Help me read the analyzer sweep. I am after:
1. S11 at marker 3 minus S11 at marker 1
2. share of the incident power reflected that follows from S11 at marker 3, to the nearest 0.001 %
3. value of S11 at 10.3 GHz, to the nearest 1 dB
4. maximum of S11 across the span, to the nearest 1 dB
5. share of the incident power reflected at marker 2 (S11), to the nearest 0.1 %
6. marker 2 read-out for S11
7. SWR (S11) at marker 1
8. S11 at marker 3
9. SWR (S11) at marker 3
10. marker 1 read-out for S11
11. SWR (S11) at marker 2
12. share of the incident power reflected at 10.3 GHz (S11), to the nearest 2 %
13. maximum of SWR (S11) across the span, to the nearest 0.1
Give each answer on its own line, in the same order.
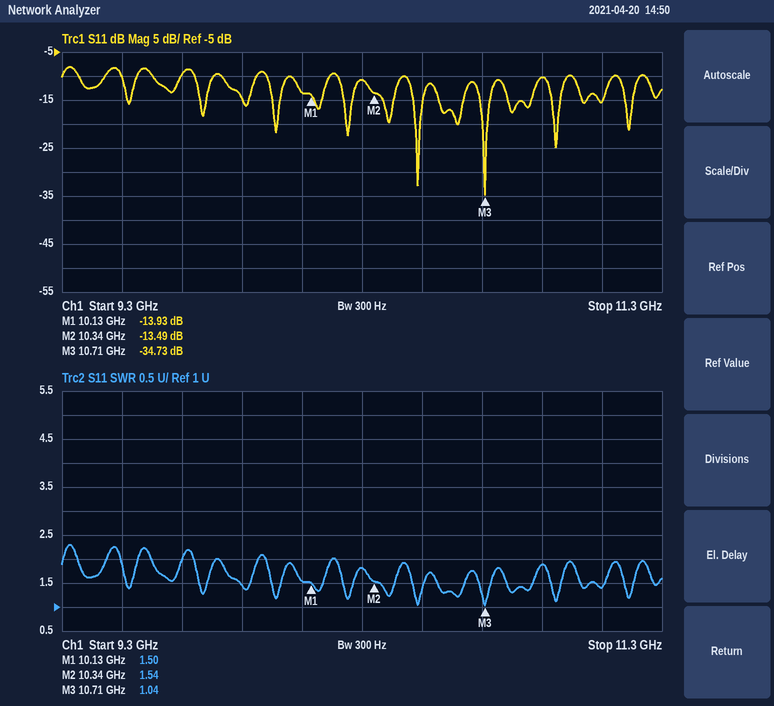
-20.80 dB
0.034 %
-11 dB
-8 dB
4.5 %
-13.49 dB
1.50
-34.73 dB
1.04
-13.93 dB
1.54
8 %
2.3
